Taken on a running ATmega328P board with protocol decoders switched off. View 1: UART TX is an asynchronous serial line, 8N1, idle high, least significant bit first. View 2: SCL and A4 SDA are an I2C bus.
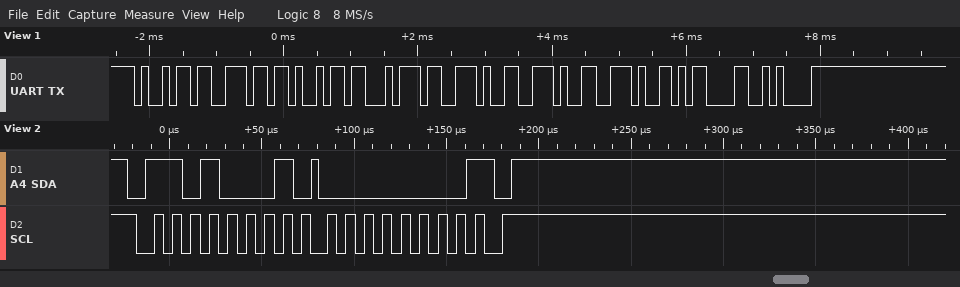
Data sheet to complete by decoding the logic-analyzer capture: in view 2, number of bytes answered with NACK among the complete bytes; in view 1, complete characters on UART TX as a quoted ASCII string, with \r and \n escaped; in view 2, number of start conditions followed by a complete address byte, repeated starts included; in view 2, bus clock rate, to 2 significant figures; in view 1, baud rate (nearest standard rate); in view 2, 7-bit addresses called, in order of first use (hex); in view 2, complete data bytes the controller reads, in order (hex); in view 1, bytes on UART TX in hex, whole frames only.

1
"init...\r\n"
1
100 kHz
9600 baud
0x68
00
0x69 0x6E 0x69 0x74 0x2E 0x2E 0x2E 0x0D 0x0A
